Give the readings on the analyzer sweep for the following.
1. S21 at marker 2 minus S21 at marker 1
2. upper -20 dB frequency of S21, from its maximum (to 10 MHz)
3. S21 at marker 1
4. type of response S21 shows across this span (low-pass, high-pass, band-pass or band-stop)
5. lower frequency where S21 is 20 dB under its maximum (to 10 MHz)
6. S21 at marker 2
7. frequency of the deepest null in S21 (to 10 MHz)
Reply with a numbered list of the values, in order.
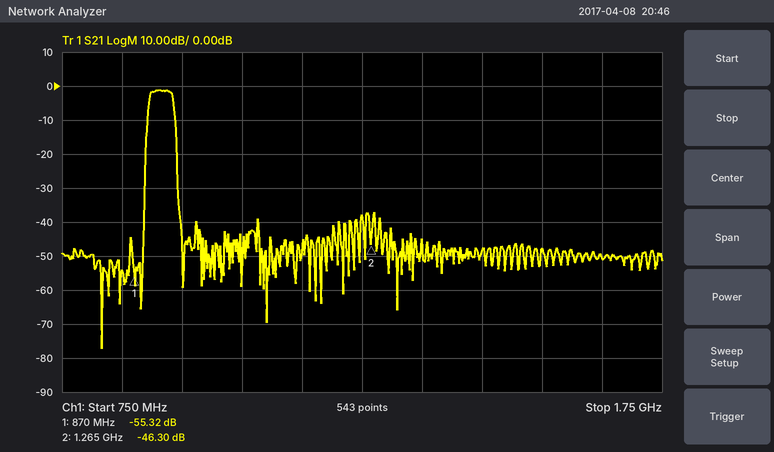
1. 9.02 dB
2. 940 MHz
3. -55.32 dB
4. band-pass
5. 890 MHz
6. -46.30 dB
7. 820 MHz
